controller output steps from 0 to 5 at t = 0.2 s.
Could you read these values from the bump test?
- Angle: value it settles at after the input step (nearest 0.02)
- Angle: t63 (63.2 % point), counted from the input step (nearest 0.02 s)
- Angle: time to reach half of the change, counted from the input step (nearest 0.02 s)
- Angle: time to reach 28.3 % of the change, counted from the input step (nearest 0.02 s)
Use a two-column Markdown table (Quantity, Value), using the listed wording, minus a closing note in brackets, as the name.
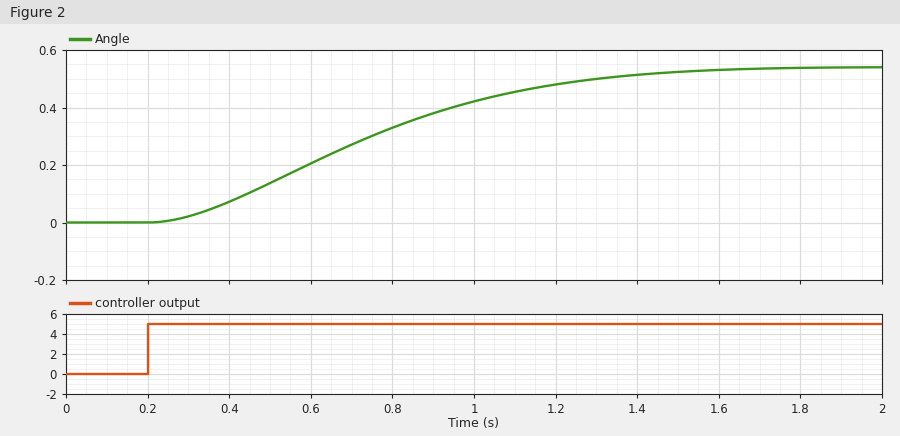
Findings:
| Quantity | Value |
|---|---|
| Angle: value it settles at after the input step | 0.54 |
| Angle: t63 (63.2 % point), counted from the input step | 0.62 s |
| Angle: time to reach half of the change, counted from the input step | 0.50 s |
| Angle: time to reach 28.3 % of the change, counted from the input step | 0.32 s |
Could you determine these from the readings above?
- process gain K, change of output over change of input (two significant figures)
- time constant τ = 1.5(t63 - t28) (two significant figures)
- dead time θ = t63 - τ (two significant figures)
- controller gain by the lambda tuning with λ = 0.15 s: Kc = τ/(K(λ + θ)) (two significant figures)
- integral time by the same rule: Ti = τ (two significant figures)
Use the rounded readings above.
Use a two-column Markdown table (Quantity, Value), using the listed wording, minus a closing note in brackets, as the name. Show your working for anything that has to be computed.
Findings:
| Quantity | Value |
|---|---|
| process gain K, change of output over change of input | (0.54 - 0) / 5 = 0.11 |
| time constant τ = 1.5(t63 - t28) | 1.5 × (0.62 - 0.32) = 0.45 s |
| dead time θ = t63 - τ | 0.62 - 0.45 = 0.17 s |
| controller gain by the lambda tuning with λ = 0.15 s: Kc = τ/(K(λ + θ)) | 0.45 / (0.11 × (0.15 + 0.17)) = 13 |
| integral time by the same rule: Ti = τ | 0.45 s |
